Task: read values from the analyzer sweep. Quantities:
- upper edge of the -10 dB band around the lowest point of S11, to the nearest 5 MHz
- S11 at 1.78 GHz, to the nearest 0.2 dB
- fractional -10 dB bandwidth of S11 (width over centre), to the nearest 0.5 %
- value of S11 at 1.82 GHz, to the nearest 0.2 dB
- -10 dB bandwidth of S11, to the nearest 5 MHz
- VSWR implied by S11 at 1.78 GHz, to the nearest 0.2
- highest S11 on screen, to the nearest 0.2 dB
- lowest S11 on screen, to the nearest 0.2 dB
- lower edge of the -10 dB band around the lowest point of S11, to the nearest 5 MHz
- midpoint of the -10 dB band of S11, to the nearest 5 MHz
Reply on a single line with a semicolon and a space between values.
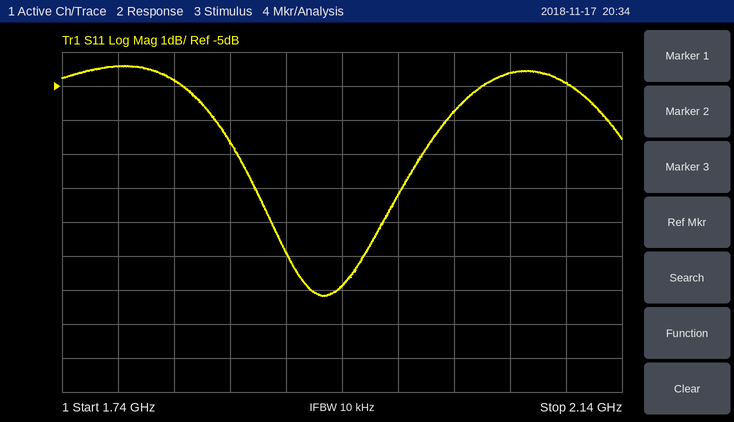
1.955 GHz; -4.4 dB; 3.0 %; -4.8 dB; 55 MHz; 4.0; -4.4 dB; -11.2 dB; 1.900 GHz; 1.930 GHz
